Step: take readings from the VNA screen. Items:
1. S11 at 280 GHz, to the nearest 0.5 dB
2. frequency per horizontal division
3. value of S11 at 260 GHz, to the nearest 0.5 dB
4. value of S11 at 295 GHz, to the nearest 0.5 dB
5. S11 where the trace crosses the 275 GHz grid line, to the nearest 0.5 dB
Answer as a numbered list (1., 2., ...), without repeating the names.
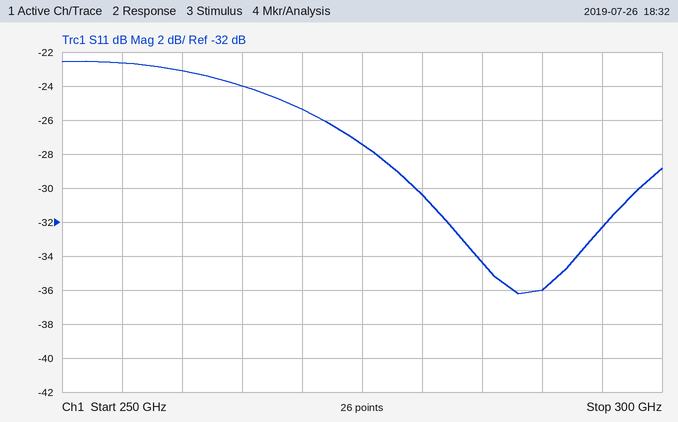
1. -30.5 dB
2. 5 GHz
3. -23.0 dB
4. -32.5 dB
5. -27.5 dB
